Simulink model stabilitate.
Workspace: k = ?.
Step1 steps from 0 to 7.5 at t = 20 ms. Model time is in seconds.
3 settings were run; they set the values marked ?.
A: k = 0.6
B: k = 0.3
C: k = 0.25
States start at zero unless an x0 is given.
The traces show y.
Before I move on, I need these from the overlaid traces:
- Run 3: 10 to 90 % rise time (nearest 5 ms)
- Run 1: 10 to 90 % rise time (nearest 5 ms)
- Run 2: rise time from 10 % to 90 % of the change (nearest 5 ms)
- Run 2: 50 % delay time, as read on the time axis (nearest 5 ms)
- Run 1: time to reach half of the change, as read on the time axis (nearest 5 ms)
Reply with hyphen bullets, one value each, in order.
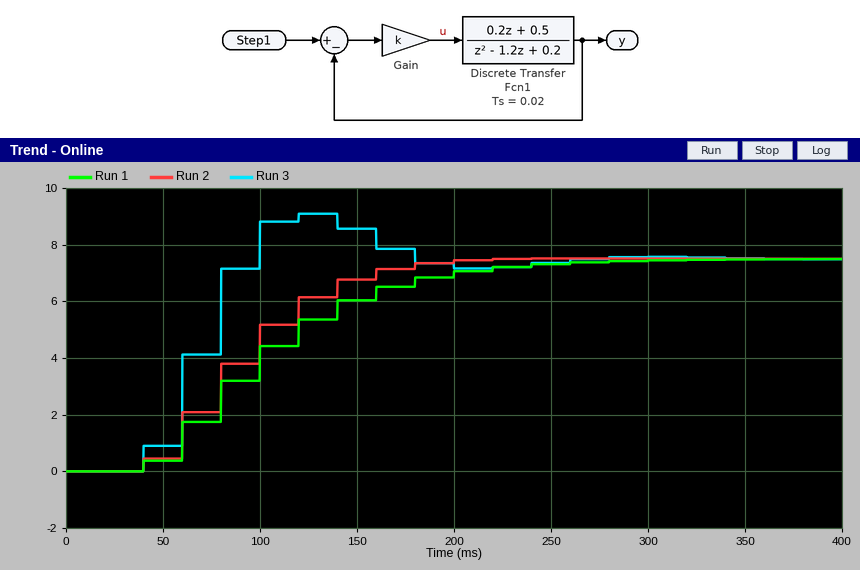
- 40 ms
- 120 ms
- 80 ms
- 80 ms
- 100 ms
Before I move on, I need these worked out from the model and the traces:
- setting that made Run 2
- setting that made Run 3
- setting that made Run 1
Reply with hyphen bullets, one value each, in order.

- B
- A
- C
